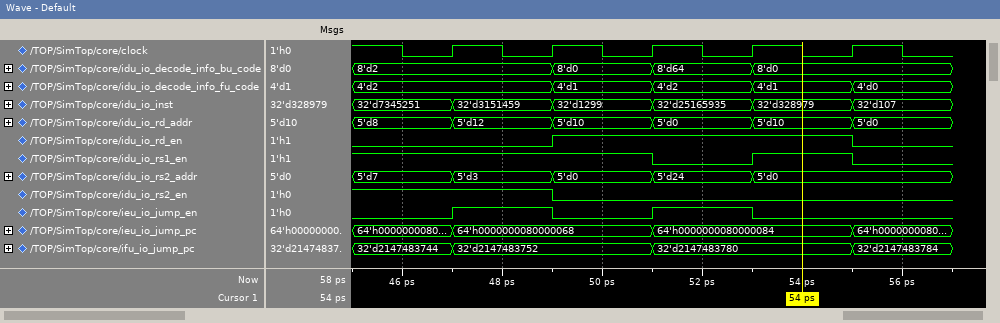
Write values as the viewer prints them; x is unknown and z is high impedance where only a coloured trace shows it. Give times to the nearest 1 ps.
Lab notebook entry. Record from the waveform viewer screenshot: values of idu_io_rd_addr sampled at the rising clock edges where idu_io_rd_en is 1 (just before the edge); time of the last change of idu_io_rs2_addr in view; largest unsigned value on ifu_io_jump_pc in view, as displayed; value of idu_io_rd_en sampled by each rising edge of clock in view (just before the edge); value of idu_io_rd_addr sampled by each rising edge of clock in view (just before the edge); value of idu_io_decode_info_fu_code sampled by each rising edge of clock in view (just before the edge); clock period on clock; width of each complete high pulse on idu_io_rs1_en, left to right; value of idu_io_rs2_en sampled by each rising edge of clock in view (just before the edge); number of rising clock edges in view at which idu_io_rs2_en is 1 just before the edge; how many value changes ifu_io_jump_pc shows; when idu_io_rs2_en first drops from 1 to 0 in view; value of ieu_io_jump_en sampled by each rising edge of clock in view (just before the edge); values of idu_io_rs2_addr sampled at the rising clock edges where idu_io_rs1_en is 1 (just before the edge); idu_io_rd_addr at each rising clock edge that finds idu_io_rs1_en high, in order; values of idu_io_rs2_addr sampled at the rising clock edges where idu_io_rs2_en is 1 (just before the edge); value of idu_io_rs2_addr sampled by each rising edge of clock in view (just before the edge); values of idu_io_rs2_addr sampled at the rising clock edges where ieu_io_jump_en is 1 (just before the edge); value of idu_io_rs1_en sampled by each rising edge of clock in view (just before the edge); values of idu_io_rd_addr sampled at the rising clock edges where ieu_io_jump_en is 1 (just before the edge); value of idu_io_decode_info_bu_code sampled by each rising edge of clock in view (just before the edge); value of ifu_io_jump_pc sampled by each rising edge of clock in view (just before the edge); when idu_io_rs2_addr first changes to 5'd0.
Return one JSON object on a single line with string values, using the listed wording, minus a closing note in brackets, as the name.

{"values of idu_io_rd_addr sampled at the rising clock edges where idu_io_rd_en is 1": "5'd10, 5'd0, 5'd10", "time of the last change of idu_io_rs2_addr in view": "53 ps", "largest unsigned value on ifu_io_jump_pc in view, as displayed": "32'd2147483784", "value of idu_io_rd_en sampled by each rising edge of clock in view": "0 0 1 1 1", "value of idu_io_rd_addr sampled by each rising edge of clock in view": "5'd8, 5'd12, 5'd10, 5'd0, 5'd10", "value of idu_io_decode_info_fu_code sampled by each rising edge of clock in view": "4'd2, 4'd2, 4'd1, 4'd2, 4'd1", "clock period on clock": "2 ps", "width of each complete high pulse on idu_io_rs1_en, left to right": "2 ps", "value of idu_io_rs2_en sampled by each rising edge of clock in view": "1 1 0 0 0", "number of rising clock edges in view at which idu_io_rs2_en is 1 just before the edge": "2", "how many value changes ifu_io_jump_pc shows": "3", "when idu_io_rs2_en first drops from 1 to 0 in view": "49 ps", "value of ieu_io_jump_en sampled by each rising edge of clock in view": "0 1 0 1 0", "values of idu_io_rs2_addr sampled at the rising clock edges where idu_io_rs1_en is 1": "5'd7, 5'd3, 5'd0, 5'd0", "idu_io_rd_addr at each rising clock edge that finds idu_io_rs1_en high, in order": "5'd8, 5'd12, 5'd10, 5'd10", "values of idu_io_rs2_addr sampled at the rising clock edges where idu_io_rs2_en is 1": "5'd7, 5'd3", "value of idu_io_rs2_addr sampled by each rising edge of clock in view": "5'd7, 5'd3, 5'd0, 5'd24, 5'd0", "values of idu_io_rs2_addr sampled at the rising clock edges where ieu_io_jump_en is 1": "5'd3, 5'd24", "value of idu_io_rs1_en sampled by each rising edge of clock in view": "1 1 1 0 1", "values of idu_io_rd_addr sampled at the rising clock edges where ieu_io_jump_en is 1": "5'd12, 5'd0", "value of idu_io_decode_info_bu_code sampled by each rising edge of clock in view": "8'd2, 8'd2, 8'd0, 8'd64, 8'd0", "value of ifu_io_jump_pc sampled by each rising edge of clock in view": "32'd2147483744, 32'd2147483752, 32'd2147483752, 32'd2147483780, 32'd2147483780", "when idu_io_rs2_addr first changes to 5'd0": "49 ps"}
